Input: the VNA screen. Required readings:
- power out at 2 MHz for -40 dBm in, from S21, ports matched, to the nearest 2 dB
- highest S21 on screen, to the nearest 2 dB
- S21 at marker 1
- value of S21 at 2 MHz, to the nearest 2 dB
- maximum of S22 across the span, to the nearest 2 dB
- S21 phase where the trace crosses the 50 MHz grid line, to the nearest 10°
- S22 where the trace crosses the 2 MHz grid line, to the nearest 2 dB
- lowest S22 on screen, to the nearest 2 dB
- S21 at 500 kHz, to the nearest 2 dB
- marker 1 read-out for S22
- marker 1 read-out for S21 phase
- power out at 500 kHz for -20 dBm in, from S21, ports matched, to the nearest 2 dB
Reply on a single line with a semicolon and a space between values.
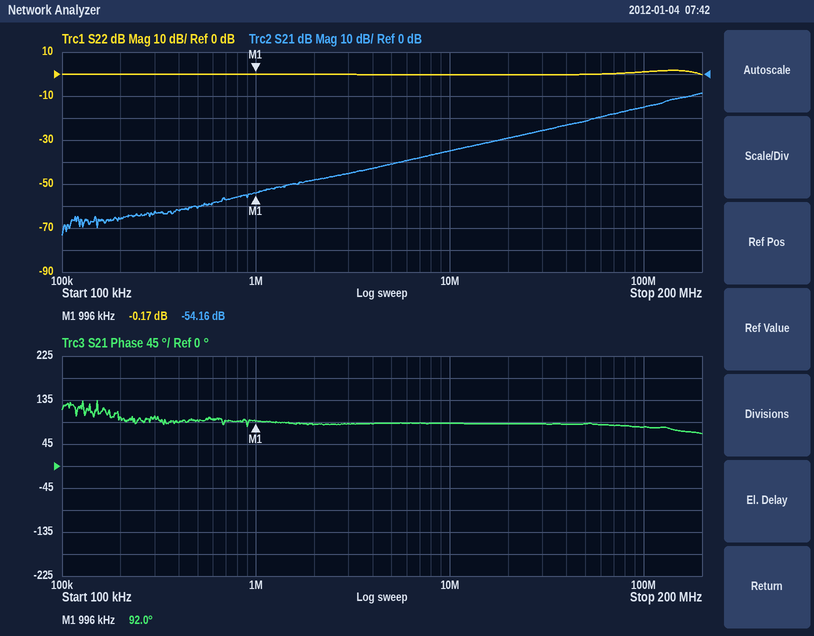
-88 dBm; -8 dB; -54.16 dB; -48 dB; 2 dB; 90°; 0 dB; 0 dB; -60 dB; -0.17 dB; 92.0°; -80 dBm
